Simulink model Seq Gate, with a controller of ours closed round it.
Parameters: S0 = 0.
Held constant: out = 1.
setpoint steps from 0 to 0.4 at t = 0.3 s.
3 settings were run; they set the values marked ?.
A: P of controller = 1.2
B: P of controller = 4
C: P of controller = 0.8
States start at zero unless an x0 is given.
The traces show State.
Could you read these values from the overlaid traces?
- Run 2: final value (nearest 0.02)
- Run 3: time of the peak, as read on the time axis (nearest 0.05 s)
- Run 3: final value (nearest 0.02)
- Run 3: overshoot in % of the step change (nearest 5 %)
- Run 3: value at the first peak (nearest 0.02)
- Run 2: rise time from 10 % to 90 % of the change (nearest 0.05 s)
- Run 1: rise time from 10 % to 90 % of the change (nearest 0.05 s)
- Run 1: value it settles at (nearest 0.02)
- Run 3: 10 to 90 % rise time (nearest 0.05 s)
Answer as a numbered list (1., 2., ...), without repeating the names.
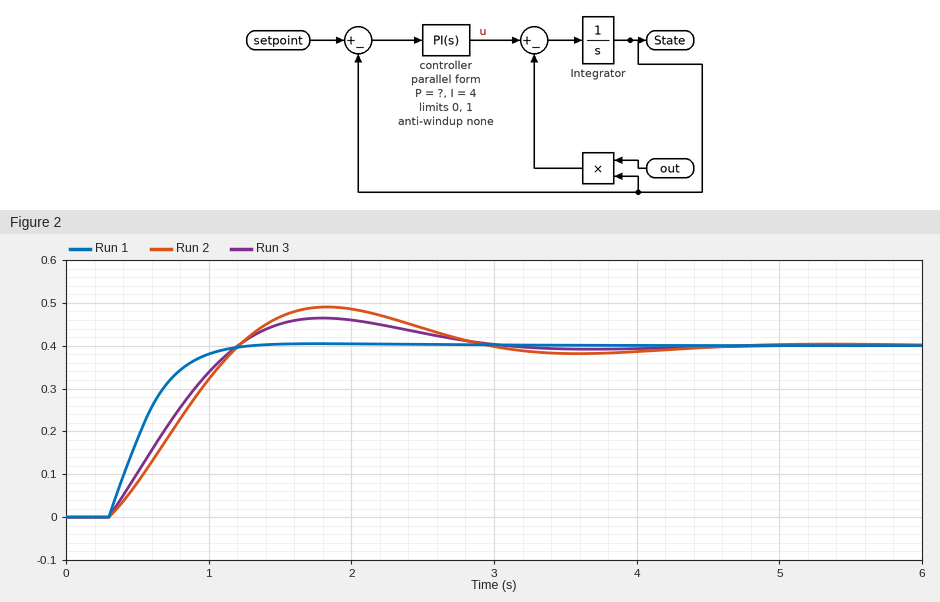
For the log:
1. 0.40
2. 1.80 s
3. 0.40
4. 15 %
5. 0.46
6. 0.70 s
7. 0.55 s
8. 0.40
9. 0.70 s
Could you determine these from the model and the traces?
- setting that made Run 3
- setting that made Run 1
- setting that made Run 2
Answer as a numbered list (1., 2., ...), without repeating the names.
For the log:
1. A
2. B
3. C
